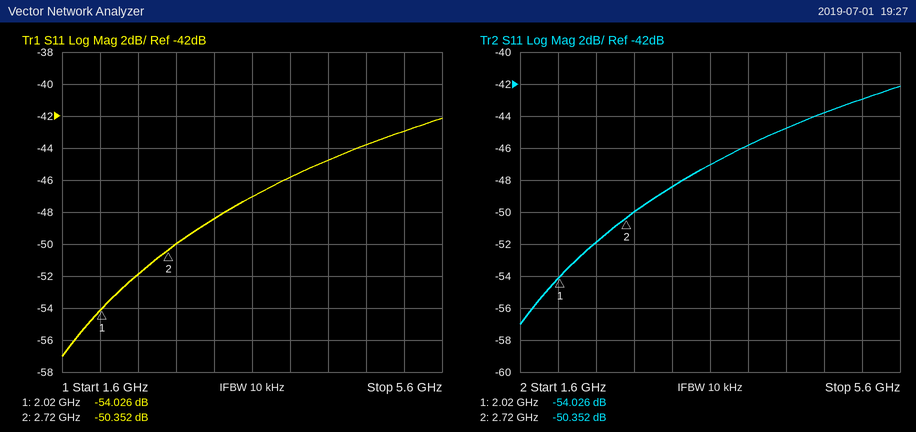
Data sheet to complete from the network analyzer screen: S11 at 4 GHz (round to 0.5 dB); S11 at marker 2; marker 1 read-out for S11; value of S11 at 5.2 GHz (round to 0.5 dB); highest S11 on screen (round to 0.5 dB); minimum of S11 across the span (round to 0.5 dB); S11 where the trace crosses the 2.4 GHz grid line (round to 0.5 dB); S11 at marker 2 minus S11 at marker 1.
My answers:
-46.0 dB
-50.352 dB
-54.026 dB
-43.0 dB
-42.0 dB
-57.0 dB
-52.0 dB
3.674 dB
